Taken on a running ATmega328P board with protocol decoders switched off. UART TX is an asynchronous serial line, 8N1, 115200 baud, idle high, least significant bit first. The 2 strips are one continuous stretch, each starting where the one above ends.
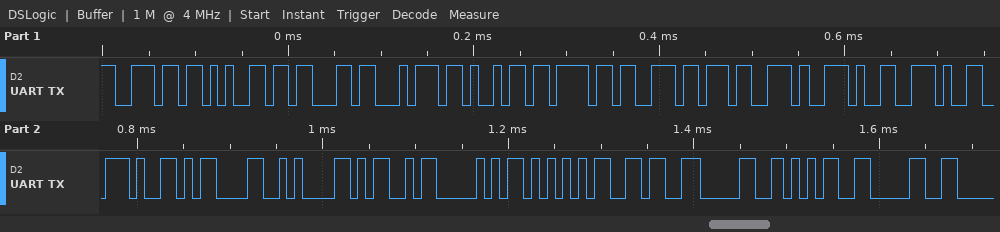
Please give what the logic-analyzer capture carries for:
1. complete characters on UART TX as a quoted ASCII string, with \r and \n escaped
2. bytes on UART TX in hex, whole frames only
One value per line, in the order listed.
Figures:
"nections...\r\nMPU6050"
6E 65 63 74 69 6F 6E 73 2E 2E 2E 0D 0A 4D 50 55 36 30 35 30
